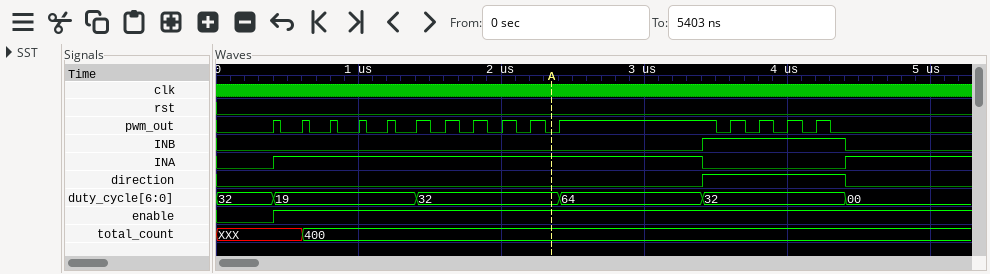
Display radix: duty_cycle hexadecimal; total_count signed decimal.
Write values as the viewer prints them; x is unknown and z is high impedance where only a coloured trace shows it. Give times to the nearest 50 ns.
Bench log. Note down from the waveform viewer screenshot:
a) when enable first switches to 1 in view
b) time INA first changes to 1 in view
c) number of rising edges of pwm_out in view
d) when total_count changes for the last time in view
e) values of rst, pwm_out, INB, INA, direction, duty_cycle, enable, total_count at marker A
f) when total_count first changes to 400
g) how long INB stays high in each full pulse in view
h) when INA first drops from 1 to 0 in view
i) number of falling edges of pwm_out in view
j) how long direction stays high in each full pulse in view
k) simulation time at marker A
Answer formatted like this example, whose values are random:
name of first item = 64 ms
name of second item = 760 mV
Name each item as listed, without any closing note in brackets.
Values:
when enable first switches to 1 in view = 400 ns
time INA first changes to 1 in view = 400 ns
number of rising edges of pwm_out in view = 15
when total_count changes for the last time in view = 600 ns
values of rst, pwm_out, INB, INA, direction, duty_cycle, enable, total_count at marker A = rst=0, pwm_out=0, INB=0, INA=1, direction=0, duty_cycle=32, enable=1, total_count=400
when total_count first changes to 400 = 600 ns
how long INB stays high in each full pulse in view = 1000 ns
when INA first drops from 1 to 0 in view = 3400 ns
number of falling edges of pwm_out in view = 15
how long direction stays high in each full pulse in view = 1000 ns
simulation time at marker A = 2350 ns
